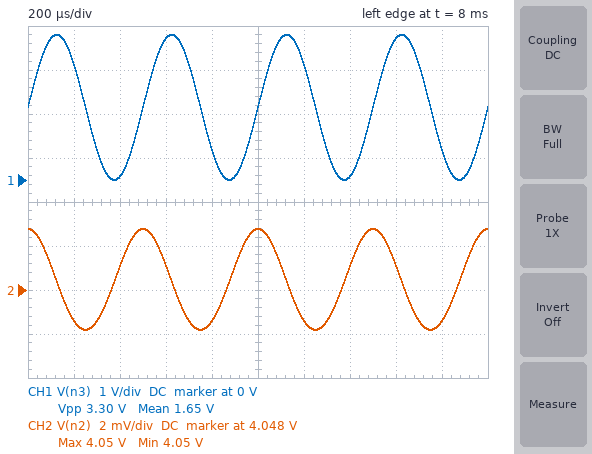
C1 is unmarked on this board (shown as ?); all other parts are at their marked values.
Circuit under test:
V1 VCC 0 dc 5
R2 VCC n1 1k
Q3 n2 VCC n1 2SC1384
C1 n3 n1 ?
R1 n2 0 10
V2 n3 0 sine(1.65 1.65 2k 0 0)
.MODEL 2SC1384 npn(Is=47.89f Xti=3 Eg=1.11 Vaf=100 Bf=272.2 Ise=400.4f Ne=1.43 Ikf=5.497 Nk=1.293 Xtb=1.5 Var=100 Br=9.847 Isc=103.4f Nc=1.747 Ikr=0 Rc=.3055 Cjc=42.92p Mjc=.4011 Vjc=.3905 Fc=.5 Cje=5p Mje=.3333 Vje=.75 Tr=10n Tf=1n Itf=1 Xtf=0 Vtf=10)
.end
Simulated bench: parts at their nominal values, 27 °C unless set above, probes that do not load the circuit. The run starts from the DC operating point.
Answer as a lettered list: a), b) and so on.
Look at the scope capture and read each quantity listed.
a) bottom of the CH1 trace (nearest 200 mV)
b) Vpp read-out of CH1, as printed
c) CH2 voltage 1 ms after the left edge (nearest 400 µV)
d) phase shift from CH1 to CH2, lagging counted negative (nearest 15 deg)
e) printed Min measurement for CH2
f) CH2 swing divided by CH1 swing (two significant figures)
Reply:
a) 0 V
b) 3.30 V
c) 4.0508 V
d) 90 deg
e) 4.05 V
f) 0.0014
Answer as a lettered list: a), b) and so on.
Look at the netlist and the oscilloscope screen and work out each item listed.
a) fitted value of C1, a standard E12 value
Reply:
a) 1.8 µF
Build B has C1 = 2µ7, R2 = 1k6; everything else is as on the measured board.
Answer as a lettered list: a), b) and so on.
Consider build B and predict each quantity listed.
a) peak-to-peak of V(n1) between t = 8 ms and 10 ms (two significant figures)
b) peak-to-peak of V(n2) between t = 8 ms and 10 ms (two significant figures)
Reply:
a) 8.9 mV
b) 6.9 mV
